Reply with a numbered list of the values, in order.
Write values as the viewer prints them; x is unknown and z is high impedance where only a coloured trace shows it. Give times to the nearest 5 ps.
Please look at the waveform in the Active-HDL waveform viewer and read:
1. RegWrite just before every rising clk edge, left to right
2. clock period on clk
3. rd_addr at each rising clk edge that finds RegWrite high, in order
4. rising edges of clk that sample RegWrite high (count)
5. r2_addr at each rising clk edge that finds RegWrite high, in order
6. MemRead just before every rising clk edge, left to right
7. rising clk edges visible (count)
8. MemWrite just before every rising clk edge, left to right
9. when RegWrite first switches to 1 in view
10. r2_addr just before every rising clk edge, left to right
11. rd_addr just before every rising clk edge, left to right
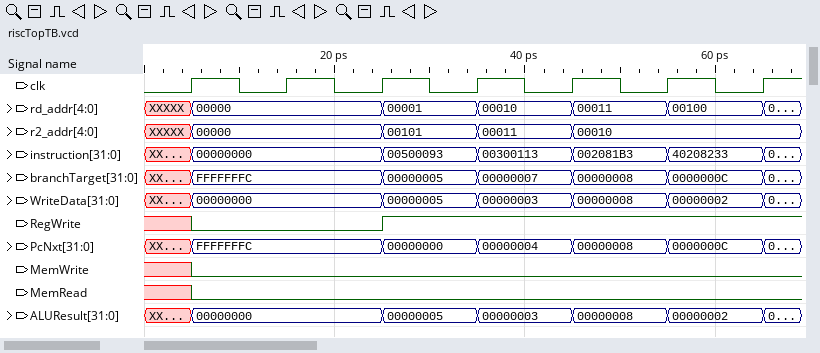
1. x 0 0 1 1 1 1
2. 10 ps
3. 00001, 00010, 00011, 00100
4. 4
5. 00101, 00011, 00010, 00010
6. x 0 0 0 0 0 0
7. 7
8. x 0 0 0 0 0 0
9. 25 ps
10. XXXXX, 00000, 00000, 00101, 00011, 00010, 00010
11. XXXXX, 00000, 00000, 00001, 00010, 00011, 00100
